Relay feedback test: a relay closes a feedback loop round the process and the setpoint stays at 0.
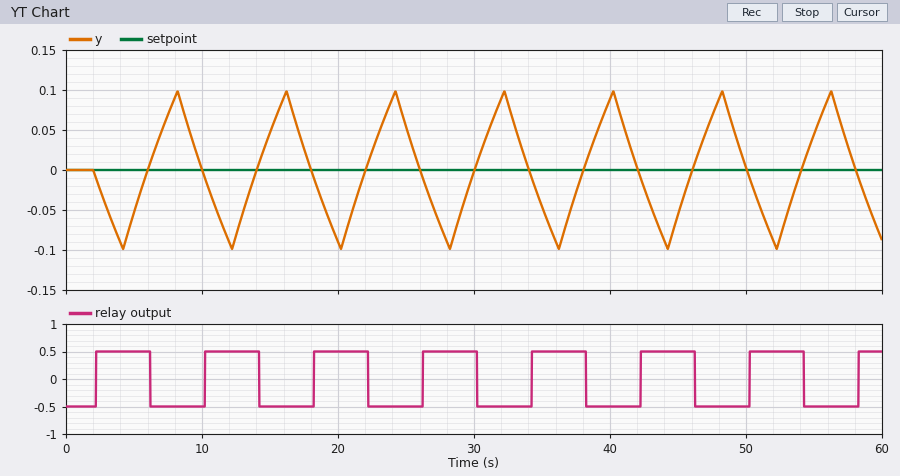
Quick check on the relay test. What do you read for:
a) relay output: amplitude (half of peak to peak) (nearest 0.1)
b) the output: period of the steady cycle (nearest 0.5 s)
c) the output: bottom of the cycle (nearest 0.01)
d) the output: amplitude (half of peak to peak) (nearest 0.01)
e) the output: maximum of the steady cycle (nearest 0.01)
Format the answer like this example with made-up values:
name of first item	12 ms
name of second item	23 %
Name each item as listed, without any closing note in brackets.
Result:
relay output: amplitude (half of peak to peak)	0.5
the output: period of the steady cycle	8.0 s
the output: bottom of the cycle	-0.10
the output: amplitude (half of peak to peak)	0.10
the output: maximum of the steady cycle	0.10
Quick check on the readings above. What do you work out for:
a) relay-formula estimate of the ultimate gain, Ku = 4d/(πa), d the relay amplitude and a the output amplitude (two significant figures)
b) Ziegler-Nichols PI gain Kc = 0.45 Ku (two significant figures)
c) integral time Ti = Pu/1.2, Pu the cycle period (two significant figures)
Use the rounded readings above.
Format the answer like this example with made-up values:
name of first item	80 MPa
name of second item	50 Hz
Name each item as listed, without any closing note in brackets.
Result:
relay-formula estimate of the ultimate gain, Ku = 4d/(πa), d the relay amplitude and a the output amplitude	6.4
Ziegler-Nichols PI gain Kc = 0.45 Ku	2.9
integral time Ti = Pu/1.2, Pu the cycle period	6.7 s
